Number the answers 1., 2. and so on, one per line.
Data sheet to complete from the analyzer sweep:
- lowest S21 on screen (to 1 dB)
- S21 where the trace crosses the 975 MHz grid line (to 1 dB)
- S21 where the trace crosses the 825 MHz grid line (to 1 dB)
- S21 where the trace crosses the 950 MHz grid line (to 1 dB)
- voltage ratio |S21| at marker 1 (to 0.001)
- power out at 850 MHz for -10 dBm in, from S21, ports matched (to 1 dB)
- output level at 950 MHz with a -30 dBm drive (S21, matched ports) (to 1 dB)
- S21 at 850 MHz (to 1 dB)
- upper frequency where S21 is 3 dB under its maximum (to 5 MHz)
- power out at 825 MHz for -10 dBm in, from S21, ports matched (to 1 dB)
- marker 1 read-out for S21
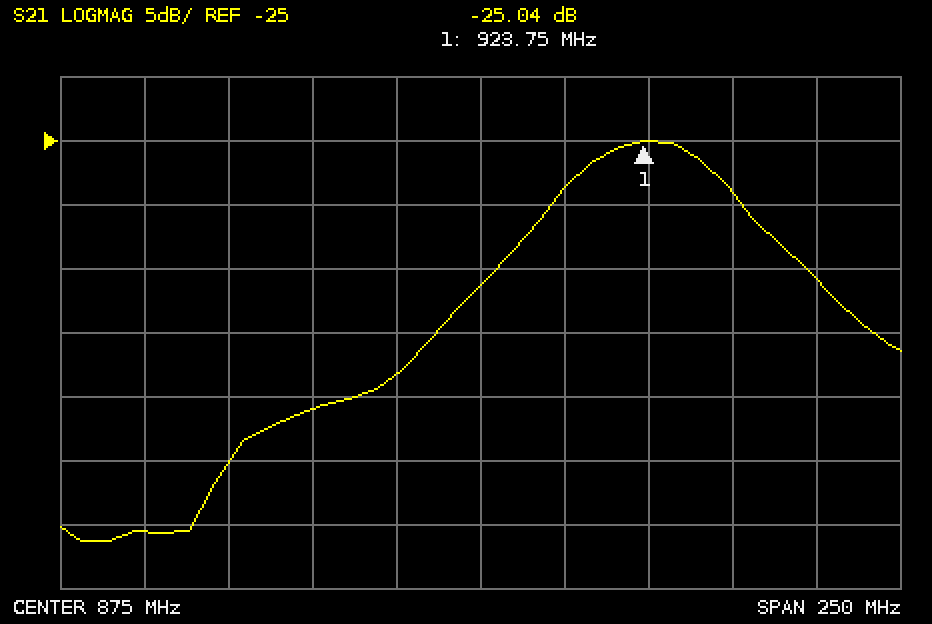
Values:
1. -56 dB
2. -36 dB
3. -46 dB
4. -29 dB
5. 0.056
6. -53 dBm
7. -59 dBm
8. -43 dB
9. 945 MHz
10. -56 dBm
11. -25.04 dB
